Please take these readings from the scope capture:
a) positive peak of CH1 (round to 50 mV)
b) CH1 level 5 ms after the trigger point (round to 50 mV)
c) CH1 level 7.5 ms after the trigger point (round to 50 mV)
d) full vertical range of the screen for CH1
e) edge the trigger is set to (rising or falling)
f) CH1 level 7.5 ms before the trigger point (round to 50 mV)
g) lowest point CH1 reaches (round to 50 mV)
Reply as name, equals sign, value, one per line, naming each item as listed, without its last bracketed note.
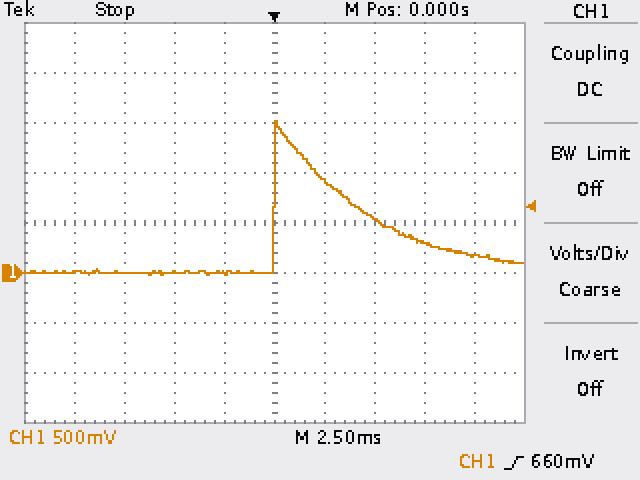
positive peak of CH1 = 1.50 V
CH1 level 5 ms after the trigger point = 550 mV
CH1 level 7.5 ms after the trigger point = 300 mV
full vertical range of the screen for CH1 = 4 V
edge the trigger is set to = rising
CH1 level 7.5 ms before the trigger point = 0 mV
lowest point CH1 reaches = 0 mV
